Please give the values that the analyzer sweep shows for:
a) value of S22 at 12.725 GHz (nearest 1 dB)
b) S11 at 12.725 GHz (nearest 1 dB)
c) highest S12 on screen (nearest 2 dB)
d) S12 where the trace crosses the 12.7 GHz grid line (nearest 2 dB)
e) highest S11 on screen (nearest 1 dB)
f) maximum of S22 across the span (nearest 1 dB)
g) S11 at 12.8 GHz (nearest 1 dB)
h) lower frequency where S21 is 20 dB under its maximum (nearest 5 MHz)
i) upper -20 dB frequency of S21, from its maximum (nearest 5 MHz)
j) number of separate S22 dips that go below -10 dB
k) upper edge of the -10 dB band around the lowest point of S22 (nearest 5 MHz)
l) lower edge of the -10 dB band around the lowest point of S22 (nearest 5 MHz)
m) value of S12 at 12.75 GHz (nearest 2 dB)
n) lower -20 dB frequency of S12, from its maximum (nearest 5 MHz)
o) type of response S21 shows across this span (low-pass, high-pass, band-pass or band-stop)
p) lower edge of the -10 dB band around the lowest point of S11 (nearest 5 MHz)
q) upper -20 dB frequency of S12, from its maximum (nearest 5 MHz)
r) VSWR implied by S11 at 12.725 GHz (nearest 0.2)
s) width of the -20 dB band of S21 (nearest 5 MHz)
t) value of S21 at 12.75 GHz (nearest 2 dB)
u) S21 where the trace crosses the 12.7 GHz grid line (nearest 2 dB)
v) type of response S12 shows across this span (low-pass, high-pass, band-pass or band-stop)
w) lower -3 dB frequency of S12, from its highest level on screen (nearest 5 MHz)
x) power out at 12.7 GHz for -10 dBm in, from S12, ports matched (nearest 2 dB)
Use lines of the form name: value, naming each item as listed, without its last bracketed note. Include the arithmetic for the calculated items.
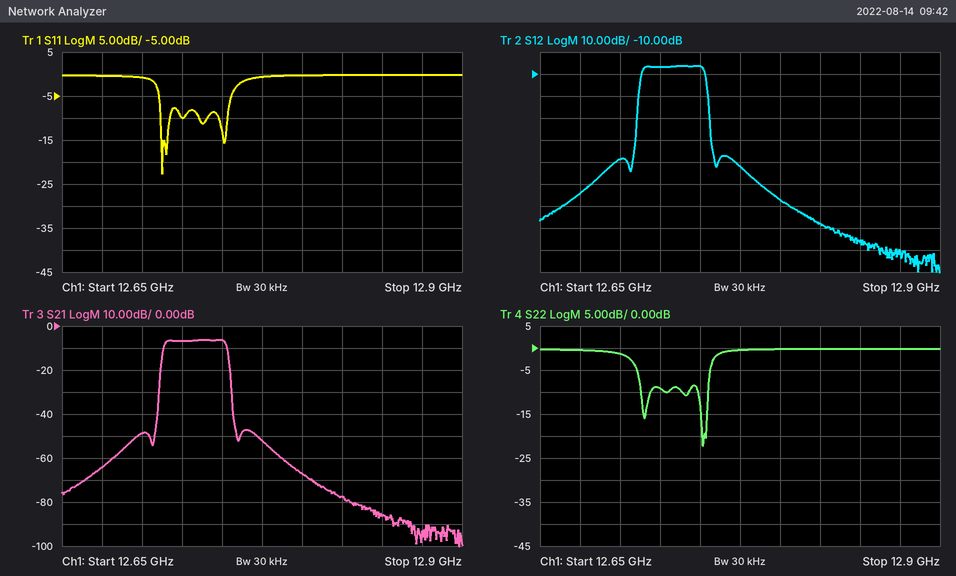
value of S22 at 12.725 GHz: -9 dB
S11 at 12.725 GHz: -10 dB
highest S12 on screen: -6 dB
S12 where the trace crosses the 12.7 GHz grid line: -48 dB
highest S11 on screen: 0 dB
maximum of S22 across the span: 0 dB
S11 at 12.8 GHz: 0 dB
lower frequency where S21 is 20 dB under its maximum: 12.710 GHz
upper -20 dB frequency of S21, from its maximum: 12.755 GHz
number of separate S22 dips that go below -10 dB: 2
upper edge of the -10 dB band around the lowest point of S22: 12.755 GHz
lower edge of the -10 dB band around the lowest point of S22: 12.750 GHz
value of S12 at 12.75 GHz: -6 dB
lower -20 dB frequency of S12, from its maximum: 12.710 GHz
type of response S21 shows across this span: band-pass
lower edge of the -10 dB band around the lowest point of S11: 12.710 GHz
upper -20 dB frequency of S12, from its maximum: 12.755 GHz
VSWR implied by S11 at 12.725 GHz: |Γ| = 10^(-10/20) = 0.3162; VSWR = (1 + 0.3162)/(1 − 0.3162) ≈ 1.92, so 2.0 to the nearest 0.2
width of the -20 dB band of S21: 12.755 GHz − 12.710 GHz = 45 MHz
value of S21 at 12.75 GHz: -6 dB
S21 where the trace crosses the 12.7 GHz grid line: -48 dB
type of response S12 shows across this span: band-pass
lower -3 dB frequency of S12, from its highest level on screen: 12.715 GHz
power out at 12.7 GHz for -10 dBm in, from S12, ports matched: -10 dBm + (-48 dB) = -58 dBm
